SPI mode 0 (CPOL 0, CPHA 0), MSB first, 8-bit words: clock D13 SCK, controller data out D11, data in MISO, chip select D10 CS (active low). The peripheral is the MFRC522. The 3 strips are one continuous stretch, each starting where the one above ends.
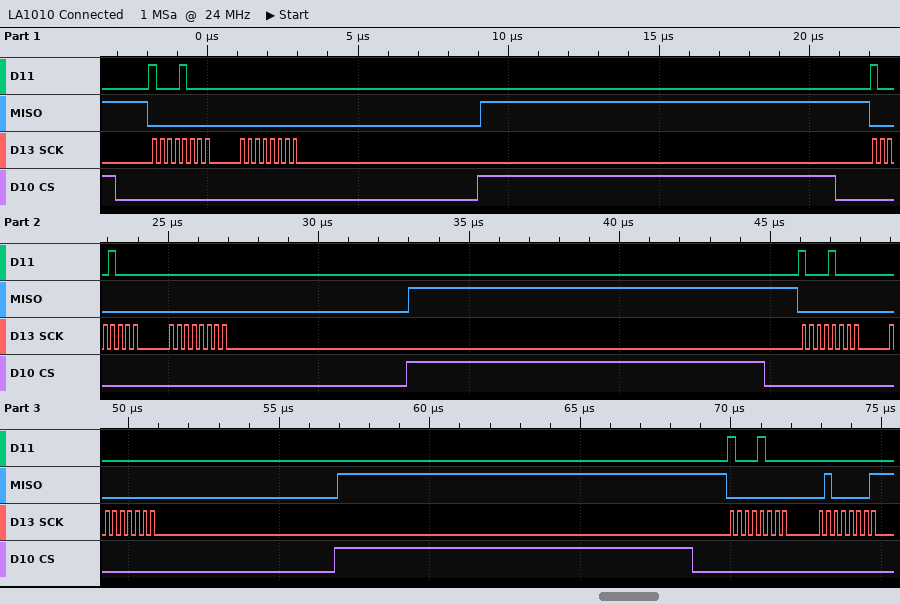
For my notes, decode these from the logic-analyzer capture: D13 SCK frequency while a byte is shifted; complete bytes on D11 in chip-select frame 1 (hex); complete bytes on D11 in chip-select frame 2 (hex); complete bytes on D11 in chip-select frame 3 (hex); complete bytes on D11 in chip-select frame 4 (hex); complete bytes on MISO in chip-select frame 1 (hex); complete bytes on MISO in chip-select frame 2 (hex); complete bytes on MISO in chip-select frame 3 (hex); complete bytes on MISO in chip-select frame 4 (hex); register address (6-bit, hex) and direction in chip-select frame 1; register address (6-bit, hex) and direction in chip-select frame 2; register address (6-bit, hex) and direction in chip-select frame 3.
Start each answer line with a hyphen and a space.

- 4 MHz
- 0x88 0x00
- 0x88 0x00
- 0x88 0x00
- 0x88 0x00
- 0x00 0x00
- 0x00 0x00
- 0x00 0x00
- 0x00 0x41
- 0x04 read
- 0x04 read
- 0x04 read
